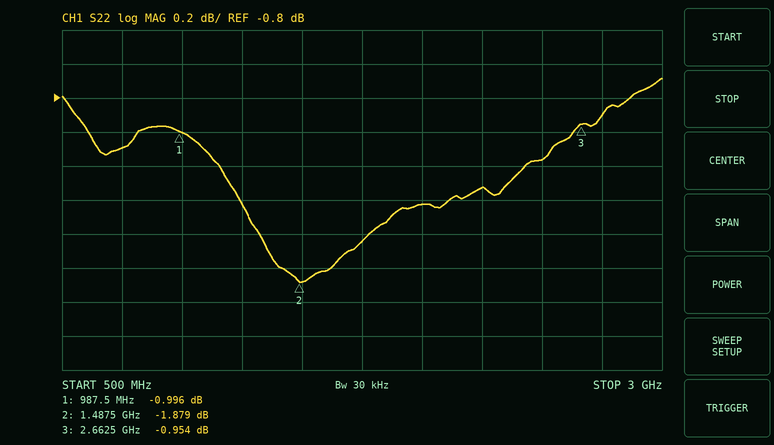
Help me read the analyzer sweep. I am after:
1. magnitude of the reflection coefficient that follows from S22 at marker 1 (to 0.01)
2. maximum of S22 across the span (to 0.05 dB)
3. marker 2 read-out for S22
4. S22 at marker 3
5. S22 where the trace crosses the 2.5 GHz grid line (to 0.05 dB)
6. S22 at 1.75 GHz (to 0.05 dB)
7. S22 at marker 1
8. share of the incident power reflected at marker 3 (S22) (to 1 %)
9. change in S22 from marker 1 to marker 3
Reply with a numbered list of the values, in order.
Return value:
1. 0.89
2. -0.70 dB
3. -1.879 dB
4. -0.954 dB
5. -1.15 dB
6. -1.65 dB
7. -0.996 dB
8. 80 %
9. 0.042 dB
